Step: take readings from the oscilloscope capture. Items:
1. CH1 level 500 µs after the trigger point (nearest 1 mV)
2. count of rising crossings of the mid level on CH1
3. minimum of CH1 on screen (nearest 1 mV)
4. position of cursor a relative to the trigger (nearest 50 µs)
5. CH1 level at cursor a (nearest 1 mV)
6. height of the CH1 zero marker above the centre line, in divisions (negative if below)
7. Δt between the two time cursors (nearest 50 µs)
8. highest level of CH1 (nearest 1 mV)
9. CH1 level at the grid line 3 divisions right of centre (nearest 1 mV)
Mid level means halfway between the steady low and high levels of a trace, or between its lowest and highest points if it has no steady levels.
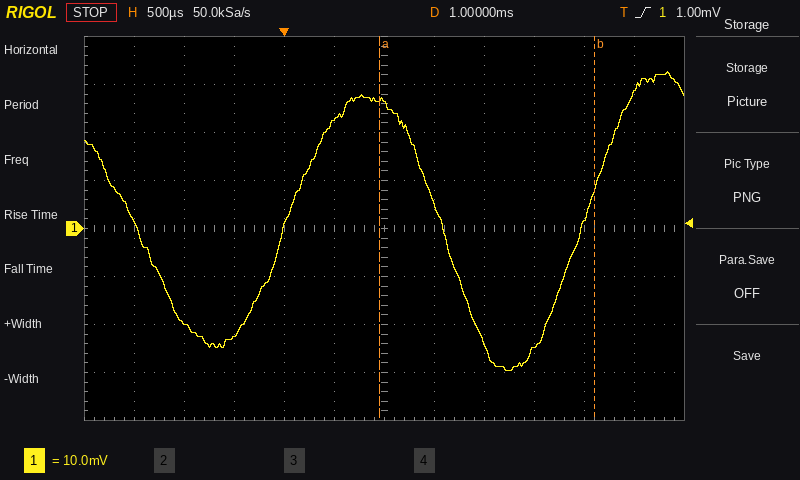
23 mV
2
-30 mV
+950 µs
27 mV
0.0 div
2.15 ms
33 mV
-25 mV
